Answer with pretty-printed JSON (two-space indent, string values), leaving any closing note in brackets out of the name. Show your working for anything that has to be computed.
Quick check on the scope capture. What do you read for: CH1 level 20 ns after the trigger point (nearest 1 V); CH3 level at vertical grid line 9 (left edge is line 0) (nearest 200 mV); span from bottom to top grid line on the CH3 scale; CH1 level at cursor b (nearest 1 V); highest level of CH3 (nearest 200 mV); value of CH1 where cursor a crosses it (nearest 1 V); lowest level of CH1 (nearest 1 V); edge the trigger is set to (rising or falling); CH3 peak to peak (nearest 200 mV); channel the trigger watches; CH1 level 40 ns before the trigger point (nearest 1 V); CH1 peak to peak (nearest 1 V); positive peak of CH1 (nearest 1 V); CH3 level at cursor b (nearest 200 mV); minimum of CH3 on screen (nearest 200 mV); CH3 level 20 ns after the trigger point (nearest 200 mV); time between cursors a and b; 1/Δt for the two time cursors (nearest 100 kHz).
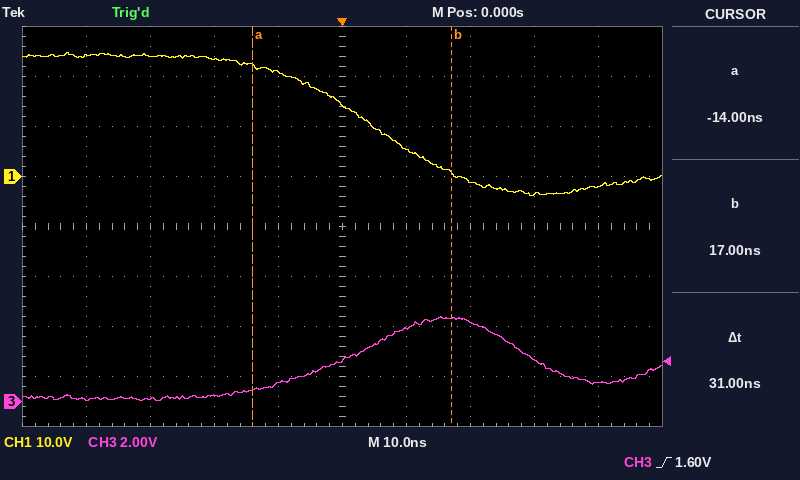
{
  "CH1 level 20 ns after the trigger point": "-1 V",
  "CH3 level at vertical grid line 9 (left edge is line 0)": "800 mV",
  "span from bottom to top grid line on the CH3 scale": "16 V",
  "CH1 level at cursor b": "1 V",
  "highest level of CH3": "3.4 V",
  "value of CH1 where cursor a crosses it": "22 V",
  "lowest level of CH1": "-4 V",
  "edge the trigger is set to": "rising",
  "CH3 peak to peak": "3.4 V − (0.0 V) = 3.4 V",
  "channel the trigger watches": "CH3",
  "CH1 level 40 ns before the trigger point": "24 V",
  "CH1 peak to peak": "25 V − (-4 V) = 29 V",
  "positive peak of CH1": "25 V",
  "CH3 level at cursor b": "3.4 V",
  "minimum of CH3 on screen": "0.0 V",
  "CH3 level 20 ns after the trigger point": "3.2 V",
  "time between cursors a and b": "31 ns",
  "1/Δt for the two time cursors": "1 / 31 ns ≈ 32.3 MHz"
}
